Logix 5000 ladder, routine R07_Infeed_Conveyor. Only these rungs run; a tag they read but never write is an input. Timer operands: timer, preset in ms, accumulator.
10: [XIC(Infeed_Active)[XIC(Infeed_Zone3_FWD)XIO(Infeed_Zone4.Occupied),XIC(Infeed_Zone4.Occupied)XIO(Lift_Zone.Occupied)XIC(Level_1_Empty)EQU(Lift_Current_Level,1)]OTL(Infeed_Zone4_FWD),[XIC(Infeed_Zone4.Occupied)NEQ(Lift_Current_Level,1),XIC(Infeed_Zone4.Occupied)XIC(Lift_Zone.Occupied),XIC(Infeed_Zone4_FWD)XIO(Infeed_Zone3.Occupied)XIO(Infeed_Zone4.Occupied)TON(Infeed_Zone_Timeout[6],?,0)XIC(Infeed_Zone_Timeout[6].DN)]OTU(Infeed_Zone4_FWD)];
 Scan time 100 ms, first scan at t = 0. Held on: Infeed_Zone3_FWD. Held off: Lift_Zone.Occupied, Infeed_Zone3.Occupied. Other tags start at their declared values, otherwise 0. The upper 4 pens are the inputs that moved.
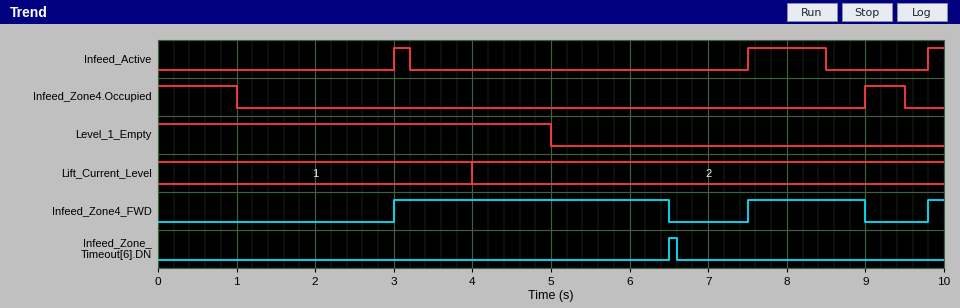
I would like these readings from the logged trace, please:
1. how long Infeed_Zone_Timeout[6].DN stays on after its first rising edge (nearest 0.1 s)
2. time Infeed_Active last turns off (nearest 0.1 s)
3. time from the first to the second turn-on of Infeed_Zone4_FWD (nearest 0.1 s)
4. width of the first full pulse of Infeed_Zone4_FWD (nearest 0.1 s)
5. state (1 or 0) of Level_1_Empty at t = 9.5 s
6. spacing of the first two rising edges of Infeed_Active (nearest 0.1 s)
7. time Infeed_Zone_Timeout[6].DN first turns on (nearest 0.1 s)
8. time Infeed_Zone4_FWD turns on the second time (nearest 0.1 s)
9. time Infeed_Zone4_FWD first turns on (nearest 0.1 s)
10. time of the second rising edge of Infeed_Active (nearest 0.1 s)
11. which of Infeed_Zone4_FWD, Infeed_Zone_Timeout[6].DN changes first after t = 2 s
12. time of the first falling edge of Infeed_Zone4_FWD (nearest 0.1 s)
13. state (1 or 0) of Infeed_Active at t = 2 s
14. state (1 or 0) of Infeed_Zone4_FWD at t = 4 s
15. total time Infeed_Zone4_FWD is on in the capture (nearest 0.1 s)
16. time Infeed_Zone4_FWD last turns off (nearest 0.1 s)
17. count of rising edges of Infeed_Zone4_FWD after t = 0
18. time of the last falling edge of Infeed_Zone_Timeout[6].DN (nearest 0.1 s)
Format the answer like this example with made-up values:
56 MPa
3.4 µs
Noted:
0.1 s
8.5 s
4.5 s
3.5 s
0
4.5 s
6.5 s
7.5 s
3.0 s
7.5 s
Infeed_Zone4_FWD
6.5 s
0
1
5.2 s
9.0 s
3
6.6 s
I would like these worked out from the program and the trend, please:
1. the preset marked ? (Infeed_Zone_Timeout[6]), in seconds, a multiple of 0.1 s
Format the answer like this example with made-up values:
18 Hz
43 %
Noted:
3.5 s
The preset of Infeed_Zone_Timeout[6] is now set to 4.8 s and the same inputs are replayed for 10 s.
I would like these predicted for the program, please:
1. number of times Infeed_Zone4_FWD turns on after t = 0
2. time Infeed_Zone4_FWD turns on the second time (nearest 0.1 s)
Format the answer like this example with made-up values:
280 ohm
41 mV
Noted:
2
9.8 s
